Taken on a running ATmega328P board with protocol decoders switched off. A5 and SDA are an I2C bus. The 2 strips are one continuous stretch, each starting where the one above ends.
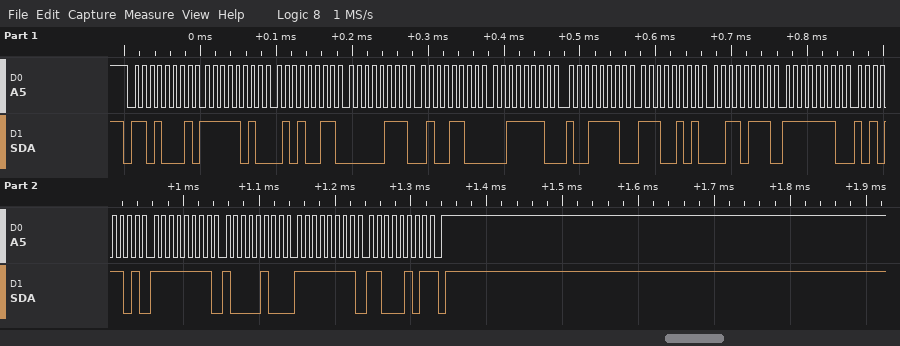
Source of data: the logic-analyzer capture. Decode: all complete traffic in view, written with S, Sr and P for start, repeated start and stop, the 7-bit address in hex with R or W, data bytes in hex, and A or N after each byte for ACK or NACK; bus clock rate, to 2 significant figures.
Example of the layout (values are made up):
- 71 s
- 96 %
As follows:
- S 68R A FA A 53 A 07 A 4C A 3E A 9E A E5 A 37 A FE A AD A FF A 84 A FF A C5 N P
- 100 kHz
